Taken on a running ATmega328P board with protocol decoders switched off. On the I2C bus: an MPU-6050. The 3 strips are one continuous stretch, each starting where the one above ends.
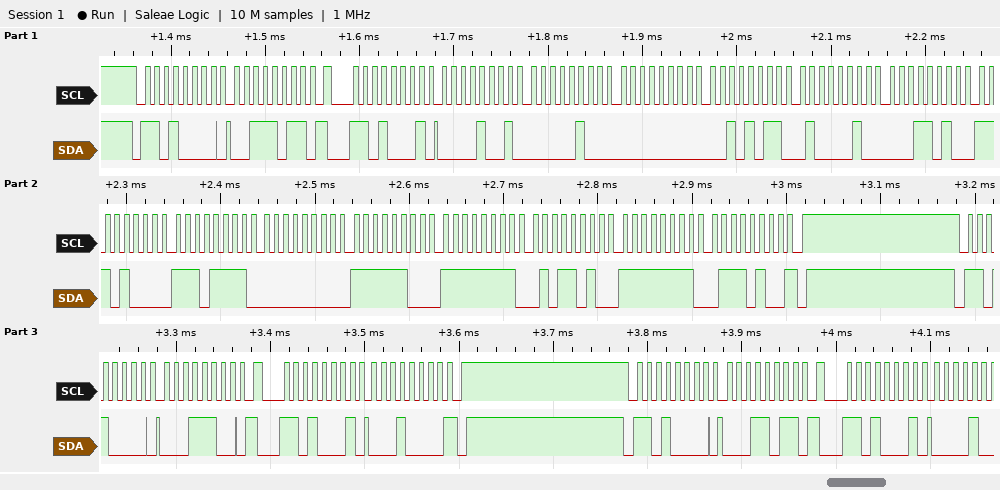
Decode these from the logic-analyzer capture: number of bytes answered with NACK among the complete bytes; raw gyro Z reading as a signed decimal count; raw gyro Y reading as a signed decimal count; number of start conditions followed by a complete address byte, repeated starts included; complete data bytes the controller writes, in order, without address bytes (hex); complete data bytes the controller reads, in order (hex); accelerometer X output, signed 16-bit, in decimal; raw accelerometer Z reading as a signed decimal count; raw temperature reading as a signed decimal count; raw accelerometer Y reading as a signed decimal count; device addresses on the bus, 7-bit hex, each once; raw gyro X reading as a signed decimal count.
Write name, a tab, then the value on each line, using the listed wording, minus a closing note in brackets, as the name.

number of bytes answered with NACK among the complete bytes	2
raw gyro Z reading as a signed decimal count	-140
raw gyro Y reading as a signed decimal count	-166
number of start conditions followed by a complete address byte, repeated starts included	6
complete data bytes the controller writes, in order, without address bytes	3B 1C 1B
complete data bytes the controller reads, in order	09 04 00 2B 42 1A E8 EF 00 FC FF 5A FF 74 10
accelerometer X output, signed 16-bit, in decimal	2308
raw accelerometer Z reading as a signed decimal count	16922
raw temperature reading as a signed decimal count	-5905
raw accelerometer Y reading as a signed decimal count	43
device addresses on the bus, 7-bit hex, each once	0x68
raw gyro X reading as a signed decimal count	252
